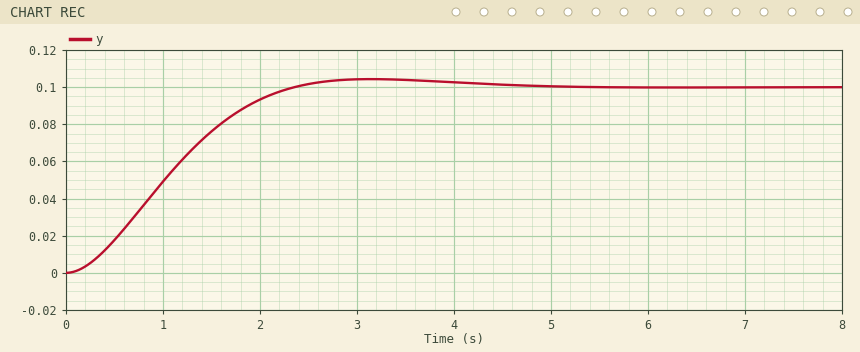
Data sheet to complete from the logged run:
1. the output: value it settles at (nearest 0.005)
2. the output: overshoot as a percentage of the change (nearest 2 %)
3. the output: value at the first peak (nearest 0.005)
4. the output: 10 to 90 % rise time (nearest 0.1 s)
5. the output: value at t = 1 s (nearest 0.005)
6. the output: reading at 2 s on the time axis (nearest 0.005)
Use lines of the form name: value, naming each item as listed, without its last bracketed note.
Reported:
the output: value it settles at: 0.100
the output: overshoot as a percentage of the change: 4 %
the output: value at the first peak: 0.105
the output: 10 to 90 % rise time: 1.5 s
the output: value at t = 1 s: 0.050
the output: reading at 2 s on the time axis: 0.095
